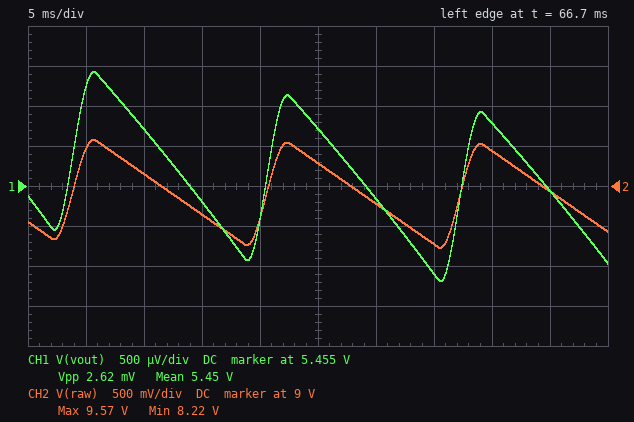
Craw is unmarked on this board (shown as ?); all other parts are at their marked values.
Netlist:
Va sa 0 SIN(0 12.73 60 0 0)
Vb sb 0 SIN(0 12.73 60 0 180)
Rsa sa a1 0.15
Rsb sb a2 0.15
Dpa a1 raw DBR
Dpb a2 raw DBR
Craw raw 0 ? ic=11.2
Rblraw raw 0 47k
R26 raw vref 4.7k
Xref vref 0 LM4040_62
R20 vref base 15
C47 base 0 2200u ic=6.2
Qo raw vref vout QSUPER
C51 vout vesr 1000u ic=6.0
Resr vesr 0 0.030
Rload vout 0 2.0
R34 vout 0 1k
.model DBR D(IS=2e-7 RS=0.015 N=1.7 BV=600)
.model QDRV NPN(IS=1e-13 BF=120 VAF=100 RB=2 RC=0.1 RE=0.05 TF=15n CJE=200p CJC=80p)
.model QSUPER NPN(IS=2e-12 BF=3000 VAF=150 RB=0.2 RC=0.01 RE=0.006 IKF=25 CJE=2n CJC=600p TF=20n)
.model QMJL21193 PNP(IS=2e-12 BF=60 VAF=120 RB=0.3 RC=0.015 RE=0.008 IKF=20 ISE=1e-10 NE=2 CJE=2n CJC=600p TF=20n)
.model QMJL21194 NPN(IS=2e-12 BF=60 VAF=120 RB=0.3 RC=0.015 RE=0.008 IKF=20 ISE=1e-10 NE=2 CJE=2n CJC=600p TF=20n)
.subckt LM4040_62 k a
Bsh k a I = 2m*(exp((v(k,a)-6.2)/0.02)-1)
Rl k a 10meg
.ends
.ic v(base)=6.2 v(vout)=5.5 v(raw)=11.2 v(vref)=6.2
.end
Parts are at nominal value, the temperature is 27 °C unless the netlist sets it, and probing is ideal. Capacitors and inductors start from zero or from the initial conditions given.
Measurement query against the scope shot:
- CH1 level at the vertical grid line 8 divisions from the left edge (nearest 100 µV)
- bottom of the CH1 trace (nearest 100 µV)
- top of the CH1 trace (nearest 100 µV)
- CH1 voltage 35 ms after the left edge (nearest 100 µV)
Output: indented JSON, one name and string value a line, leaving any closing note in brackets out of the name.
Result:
{
  "CH1 level at the vertical grid line 8 divisions from the left edge": "5.4553 V",
  "bottom of the CH1 trace": "5.4533 V",
  "top of the CH1 trace": "5.4559 V",
  "CH1 voltage 35 ms after the left edge": "5.4534 V"
}
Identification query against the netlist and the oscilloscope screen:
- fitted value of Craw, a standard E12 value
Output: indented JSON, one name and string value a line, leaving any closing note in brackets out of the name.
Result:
{
  "fitted value of Craw, a standard E12 value": "27 mF"
}
